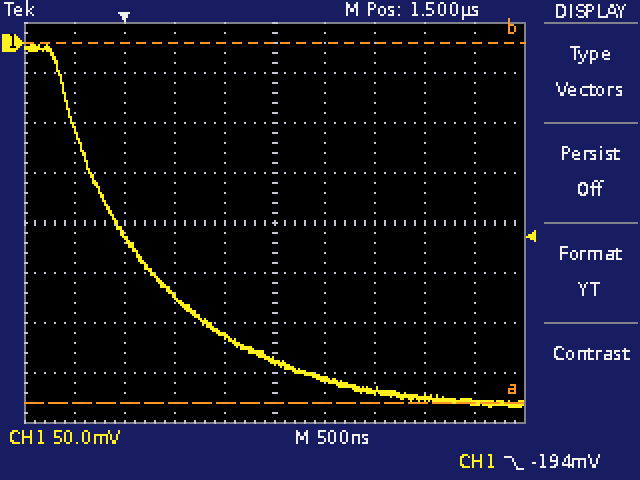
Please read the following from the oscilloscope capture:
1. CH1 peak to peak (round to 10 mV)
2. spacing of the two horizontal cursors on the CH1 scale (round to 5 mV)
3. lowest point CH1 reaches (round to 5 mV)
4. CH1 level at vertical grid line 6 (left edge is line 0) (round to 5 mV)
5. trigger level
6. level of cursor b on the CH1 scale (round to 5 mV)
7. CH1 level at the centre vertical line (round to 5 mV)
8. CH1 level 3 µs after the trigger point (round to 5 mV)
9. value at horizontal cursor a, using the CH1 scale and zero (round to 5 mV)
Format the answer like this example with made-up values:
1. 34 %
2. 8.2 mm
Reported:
1. 360 mV
2. 360 mV
3. -365 mV
4. -335 mV
5. -194 mV
6. 0 mV
7. -320 mV
8. -355 mV
9. -360 mV
